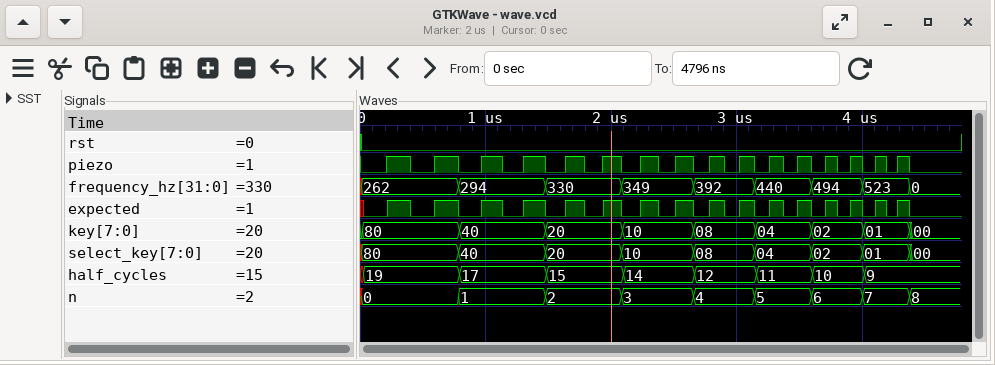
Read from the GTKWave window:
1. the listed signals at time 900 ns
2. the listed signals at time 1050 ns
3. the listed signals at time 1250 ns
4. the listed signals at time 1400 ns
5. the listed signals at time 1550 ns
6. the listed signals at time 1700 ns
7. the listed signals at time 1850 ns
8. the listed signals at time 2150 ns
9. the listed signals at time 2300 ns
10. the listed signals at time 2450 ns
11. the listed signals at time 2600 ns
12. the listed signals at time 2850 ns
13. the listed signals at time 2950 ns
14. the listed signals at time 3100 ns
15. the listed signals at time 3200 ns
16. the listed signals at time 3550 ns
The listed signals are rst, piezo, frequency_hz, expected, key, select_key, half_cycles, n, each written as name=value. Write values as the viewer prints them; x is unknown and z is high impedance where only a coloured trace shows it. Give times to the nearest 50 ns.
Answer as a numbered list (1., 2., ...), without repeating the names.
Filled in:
1. rst=0, piezo=0, frequency_hz=294, expected=0, key=40, select_key=40, half_cycles=17, n=1
2. rst=0, piezo=1, frequency_hz=294, expected=1, key=40, select_key=40, half_cycles=17, n=1
3. rst=0, piezo=0, frequency_hz=294, expected=0, key=40, select_key=40, half_cycles=17, n=1
4. rst=0, piezo=1, frequency_hz=294, expected=1, key=40, select_key=40, half_cycles=17, n=1
5. rst=0, piezo=0, frequency_hz=330, expected=0, key=20, select_key=20, half_cycles=15, n=2
6. rst=0, piezo=1, frequency_hz=330, expected=1, key=20, select_key=20, half_cycles=15, n=2
7. rst=0, piezo=0, frequency_hz=330, expected=0, key=20, select_key=20, half_cycles=15, n=2
8. rst=0, piezo=0, frequency_hz=349, expected=0, key=10, select_key=10, half_cycles=14, n=3
9. rst=0, piezo=1, frequency_hz=349, expected=1, key=10, select_key=10, half_cycles=14, n=3
10. rst=0, piezo=0, frequency_hz=349, expected=0, key=10, select_key=10, half_cycles=14, n=3
11. rst=0, piezo=1, frequency_hz=349, expected=1, key=10, select_key=10, half_cycles=14, n=3
12. rst=0, piezo=1, frequency_hz=392, expected=1, key=08, select_key=08, half_cycles=12, n=4
13. rst=0, piezo=0, frequency_hz=392, expected=0, key=08, select_key=08, half_cycles=12, n=4
14. rst=0, piezo=1, frequency_hz=392, expected=1, key=08, select_key=08, half_cycles=12, n=4
15. rst=0, piezo=0, frequency_hz=440, expected=0, key=04, select_key=04, half_cycles=11, n=5
16. rst=0, piezo=1, frequency_hz=440, expected=1, key=04, select_key=04, half_cycles=11, n=5
